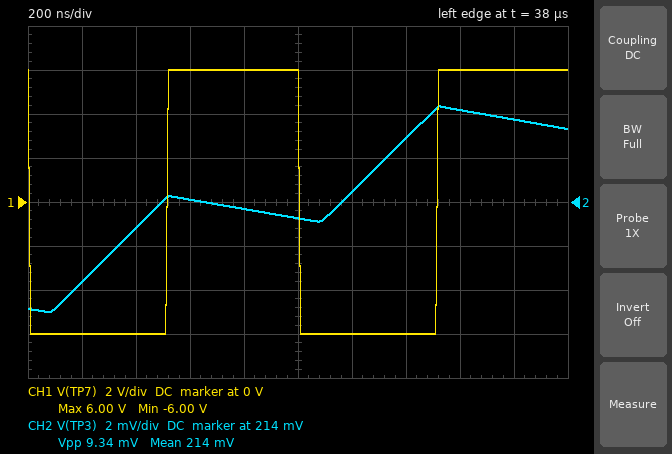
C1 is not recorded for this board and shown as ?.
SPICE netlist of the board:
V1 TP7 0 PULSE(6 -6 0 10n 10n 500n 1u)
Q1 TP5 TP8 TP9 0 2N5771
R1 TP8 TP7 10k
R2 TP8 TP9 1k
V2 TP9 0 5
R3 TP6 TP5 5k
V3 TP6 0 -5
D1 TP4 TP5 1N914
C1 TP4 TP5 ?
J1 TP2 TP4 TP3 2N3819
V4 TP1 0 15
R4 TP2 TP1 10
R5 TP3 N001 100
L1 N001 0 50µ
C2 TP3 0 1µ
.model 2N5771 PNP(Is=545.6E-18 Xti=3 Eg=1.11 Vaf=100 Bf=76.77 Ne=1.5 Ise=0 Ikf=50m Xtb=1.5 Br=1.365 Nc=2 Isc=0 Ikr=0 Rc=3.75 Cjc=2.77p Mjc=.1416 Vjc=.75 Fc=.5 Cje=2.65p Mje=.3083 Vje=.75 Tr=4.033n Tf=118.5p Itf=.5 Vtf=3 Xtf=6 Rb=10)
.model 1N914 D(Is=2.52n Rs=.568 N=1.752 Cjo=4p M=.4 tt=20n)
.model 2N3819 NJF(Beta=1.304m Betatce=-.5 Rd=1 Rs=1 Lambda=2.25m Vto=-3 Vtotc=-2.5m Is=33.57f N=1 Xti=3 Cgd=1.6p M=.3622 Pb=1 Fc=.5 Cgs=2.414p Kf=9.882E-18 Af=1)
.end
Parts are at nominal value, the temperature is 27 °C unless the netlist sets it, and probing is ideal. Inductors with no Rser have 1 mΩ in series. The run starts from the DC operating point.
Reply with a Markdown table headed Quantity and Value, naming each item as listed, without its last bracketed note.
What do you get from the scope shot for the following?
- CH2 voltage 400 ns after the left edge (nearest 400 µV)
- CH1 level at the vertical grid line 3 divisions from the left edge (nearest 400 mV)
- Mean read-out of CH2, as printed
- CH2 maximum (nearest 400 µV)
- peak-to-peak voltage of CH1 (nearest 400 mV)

| Quantity | Value |
|---|---|
| CH2 voltage 400 ns after the left edge | 212.8 mV |
| CH1 level at the vertical grid line 3 divisions from the left edge | 6.0 V |
| Mean read-out of CH2, as printed | 214 mV |
| CH2 maximum | 218.4 mV |
| peak-to-peak voltage of CH1 | 12.0 V |
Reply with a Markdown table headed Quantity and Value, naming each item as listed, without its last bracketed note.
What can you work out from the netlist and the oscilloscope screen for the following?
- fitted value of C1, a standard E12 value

| Quantity | Value |
|---|---|
| fitted value of C1, a standard E12 value | 100 pF |
